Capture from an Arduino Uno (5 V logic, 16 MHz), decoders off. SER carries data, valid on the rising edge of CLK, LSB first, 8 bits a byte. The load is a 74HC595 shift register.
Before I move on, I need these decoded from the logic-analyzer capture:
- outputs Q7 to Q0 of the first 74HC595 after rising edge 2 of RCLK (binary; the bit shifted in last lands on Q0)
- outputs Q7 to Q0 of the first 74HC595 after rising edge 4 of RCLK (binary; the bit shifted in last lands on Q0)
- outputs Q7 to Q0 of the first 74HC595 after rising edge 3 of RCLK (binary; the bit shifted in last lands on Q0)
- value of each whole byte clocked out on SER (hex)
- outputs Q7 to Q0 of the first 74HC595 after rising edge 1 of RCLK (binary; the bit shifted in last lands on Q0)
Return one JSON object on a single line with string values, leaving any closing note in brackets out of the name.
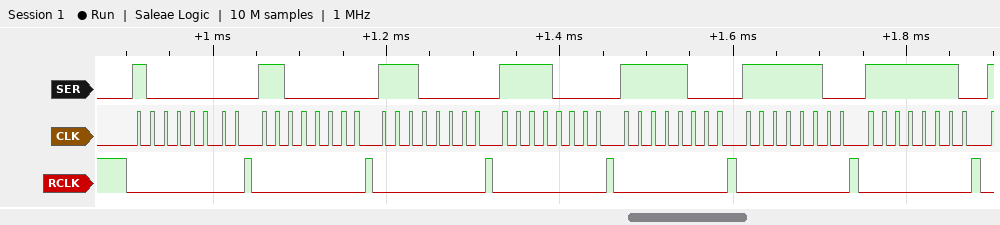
{"outputs Q7 to Q0 of the first 74HC595 after rising edge 2 of RCLK": "11000000", "outputs Q7 to Q0 of the first 74HC595 after rising edge 4 of RCLK": "11110000", "outputs Q7 to Q0 of the first 74HC595 after rising edge 3 of RCLK": "11100000", "value of each whole byte clocked out on SER": "01 03 07 0F 1F 3F 7F", "outputs Q7 to Q0 of the first 74HC595 after rising edge 1 of RCLK": "10000000"}
